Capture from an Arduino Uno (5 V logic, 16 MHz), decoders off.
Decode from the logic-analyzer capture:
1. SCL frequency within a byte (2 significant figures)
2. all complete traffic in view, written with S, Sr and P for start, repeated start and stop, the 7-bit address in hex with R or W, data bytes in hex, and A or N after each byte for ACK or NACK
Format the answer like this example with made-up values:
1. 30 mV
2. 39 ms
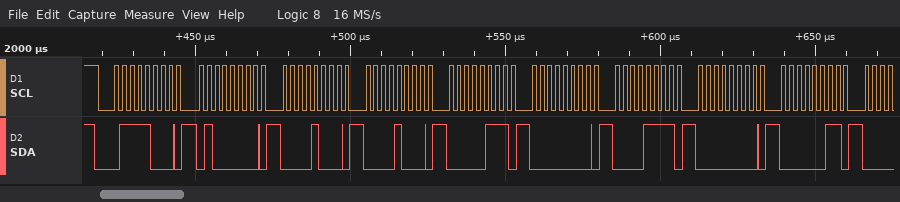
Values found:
1. 400 kHz
2. S 3CW A 40 A 08 A 08 A 07 A 00 A 0F A 00 A 03 A
